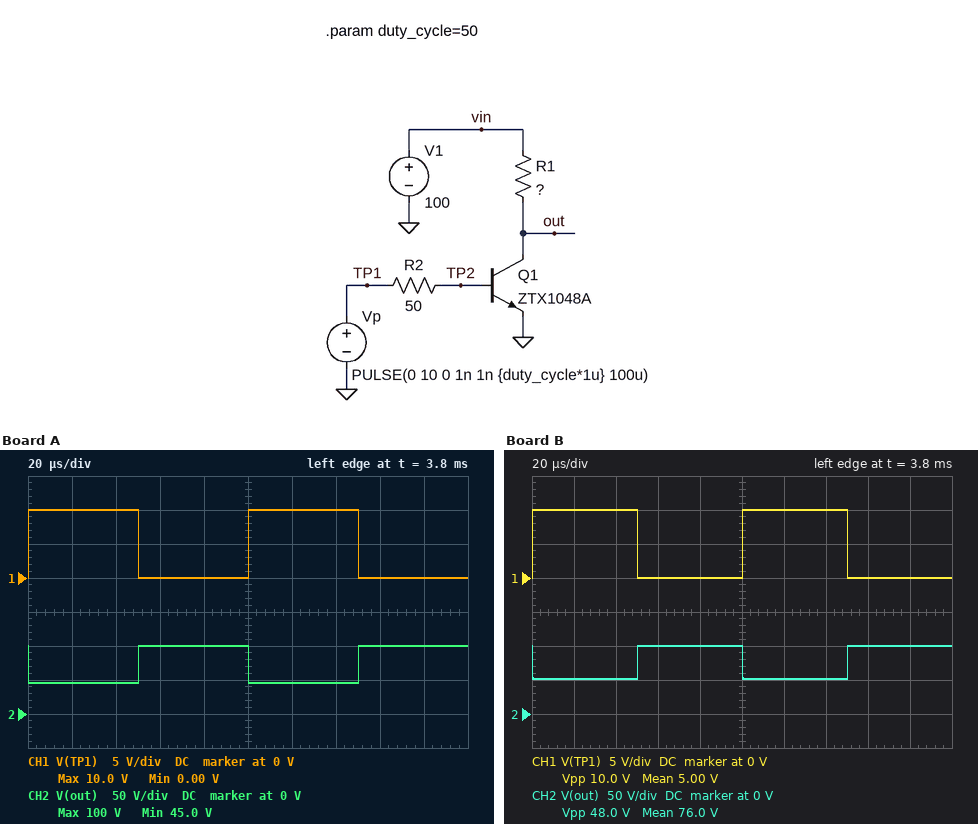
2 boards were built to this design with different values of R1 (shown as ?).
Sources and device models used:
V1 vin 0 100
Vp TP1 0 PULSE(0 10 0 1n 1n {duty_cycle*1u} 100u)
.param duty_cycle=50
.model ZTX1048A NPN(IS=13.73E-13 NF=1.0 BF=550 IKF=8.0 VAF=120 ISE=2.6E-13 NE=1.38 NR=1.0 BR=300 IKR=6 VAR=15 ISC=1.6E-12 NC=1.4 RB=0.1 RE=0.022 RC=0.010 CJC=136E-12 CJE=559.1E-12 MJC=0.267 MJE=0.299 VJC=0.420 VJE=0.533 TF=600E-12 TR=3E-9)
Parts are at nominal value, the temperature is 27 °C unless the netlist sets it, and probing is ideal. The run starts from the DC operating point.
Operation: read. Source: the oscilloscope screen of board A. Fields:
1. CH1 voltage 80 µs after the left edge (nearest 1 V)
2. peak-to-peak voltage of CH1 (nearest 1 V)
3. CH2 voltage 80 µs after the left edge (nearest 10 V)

0 V
10 V
100 V
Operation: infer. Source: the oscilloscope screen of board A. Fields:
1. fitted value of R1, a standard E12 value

1.8 Ω
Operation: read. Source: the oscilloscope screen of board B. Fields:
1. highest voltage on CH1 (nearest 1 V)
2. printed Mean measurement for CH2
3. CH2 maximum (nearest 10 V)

10 V
76.0 V
100 V
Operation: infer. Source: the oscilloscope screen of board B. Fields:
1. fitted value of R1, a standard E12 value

1.5 Ω
